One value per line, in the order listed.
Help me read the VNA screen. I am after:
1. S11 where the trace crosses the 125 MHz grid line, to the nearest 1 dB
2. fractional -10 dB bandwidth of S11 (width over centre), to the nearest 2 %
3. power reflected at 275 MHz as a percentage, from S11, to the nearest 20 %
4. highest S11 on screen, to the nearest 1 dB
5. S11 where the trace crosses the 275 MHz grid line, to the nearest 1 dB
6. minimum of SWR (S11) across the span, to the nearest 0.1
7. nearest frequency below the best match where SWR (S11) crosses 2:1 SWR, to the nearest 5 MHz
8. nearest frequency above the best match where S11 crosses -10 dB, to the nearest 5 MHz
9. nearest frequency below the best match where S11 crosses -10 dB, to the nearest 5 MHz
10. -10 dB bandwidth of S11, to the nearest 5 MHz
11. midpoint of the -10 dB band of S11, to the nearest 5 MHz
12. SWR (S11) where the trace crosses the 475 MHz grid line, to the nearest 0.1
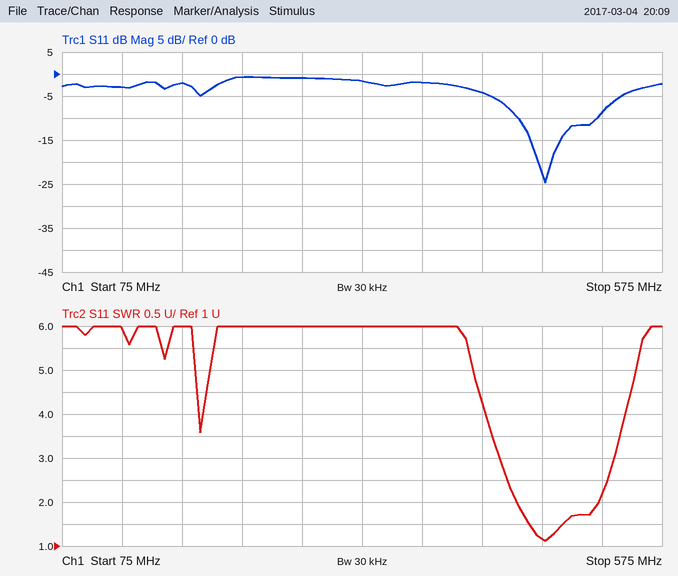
-3 dB
14 %
80 %
-1 dB
-1 dB
1.1
455 MHz
520 MHz
455 MHz
65 MHz
490 MHz
1.2
